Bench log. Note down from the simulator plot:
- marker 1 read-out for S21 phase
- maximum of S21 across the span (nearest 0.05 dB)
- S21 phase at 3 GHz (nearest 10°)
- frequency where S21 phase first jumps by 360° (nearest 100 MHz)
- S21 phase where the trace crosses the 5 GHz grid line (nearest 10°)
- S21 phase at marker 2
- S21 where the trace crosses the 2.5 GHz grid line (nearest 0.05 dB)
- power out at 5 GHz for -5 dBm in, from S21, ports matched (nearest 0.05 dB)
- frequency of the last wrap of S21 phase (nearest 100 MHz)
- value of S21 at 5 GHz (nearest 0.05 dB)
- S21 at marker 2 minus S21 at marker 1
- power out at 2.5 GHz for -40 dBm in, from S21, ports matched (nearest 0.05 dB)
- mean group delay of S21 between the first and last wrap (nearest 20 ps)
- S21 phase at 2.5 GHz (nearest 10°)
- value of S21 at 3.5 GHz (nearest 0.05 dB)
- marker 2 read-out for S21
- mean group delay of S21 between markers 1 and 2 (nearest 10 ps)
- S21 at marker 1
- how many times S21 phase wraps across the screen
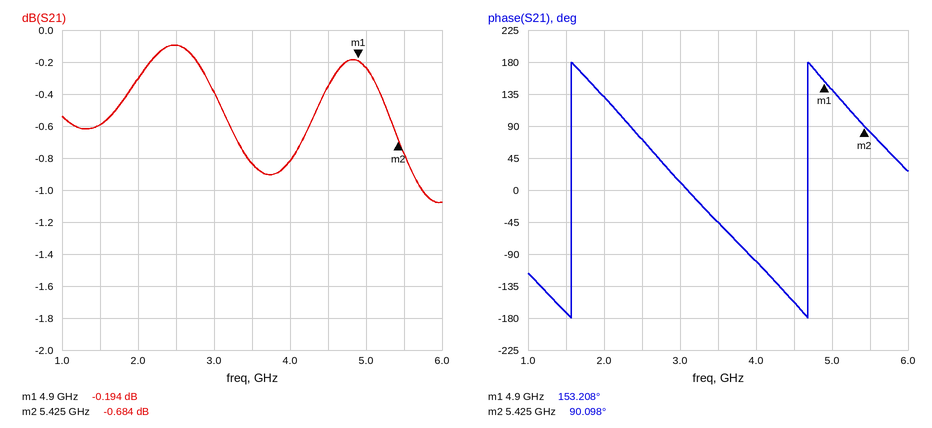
153.208°
-0.10 dB
10°
1.6 GHz
140°
90.098°
-0.10 dB
-5.25 dBm
4.7 GHz
-0.25 dB
-0.490 dB
-40.10 dBm
320 ps
70°
-0.85 dB
-0.684 dB
330 ps
-0.194 dB
2
